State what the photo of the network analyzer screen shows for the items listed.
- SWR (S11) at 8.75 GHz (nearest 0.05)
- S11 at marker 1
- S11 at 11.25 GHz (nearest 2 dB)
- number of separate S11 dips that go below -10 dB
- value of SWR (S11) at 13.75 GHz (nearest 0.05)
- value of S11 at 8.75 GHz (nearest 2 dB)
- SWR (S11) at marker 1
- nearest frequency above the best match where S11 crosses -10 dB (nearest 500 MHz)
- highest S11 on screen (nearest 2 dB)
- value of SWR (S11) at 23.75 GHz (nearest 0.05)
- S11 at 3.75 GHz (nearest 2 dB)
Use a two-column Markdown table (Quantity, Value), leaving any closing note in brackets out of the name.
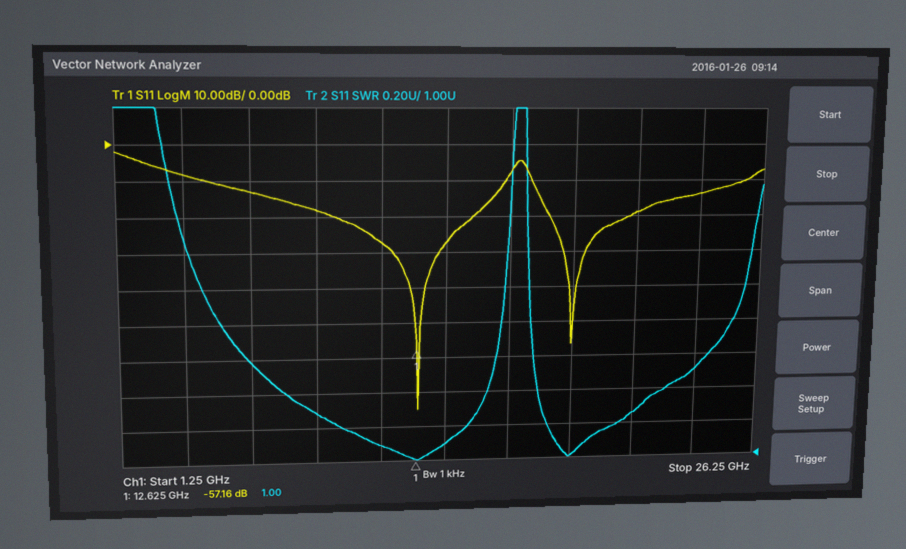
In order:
| Quantity | Value |
|---|---|
| SWR (S11) at 8.75 GHz | 1.30 |
| S11 at marker 1 | -57.16 dB |
| S11 at 11.25 GHz | -28 dB |
| number of separate S11 dips that go below -10 dB | 2 |
| value of SWR (S11) at 13.75 GHz | 1.10 |
| value of S11 at 8.75 GHz | -18 dB |
| SWR (S11) at marker 1 | 1.00 |
| nearest frequency above the best match where S11 crosses -10 dB | 16.0 GHz |
| highest S11 on screen | -2 dB |
| value of SWR (S11) at 23.75 GHz | 1.50 |
| S11 at 3.75 GHz | -8 dB |
